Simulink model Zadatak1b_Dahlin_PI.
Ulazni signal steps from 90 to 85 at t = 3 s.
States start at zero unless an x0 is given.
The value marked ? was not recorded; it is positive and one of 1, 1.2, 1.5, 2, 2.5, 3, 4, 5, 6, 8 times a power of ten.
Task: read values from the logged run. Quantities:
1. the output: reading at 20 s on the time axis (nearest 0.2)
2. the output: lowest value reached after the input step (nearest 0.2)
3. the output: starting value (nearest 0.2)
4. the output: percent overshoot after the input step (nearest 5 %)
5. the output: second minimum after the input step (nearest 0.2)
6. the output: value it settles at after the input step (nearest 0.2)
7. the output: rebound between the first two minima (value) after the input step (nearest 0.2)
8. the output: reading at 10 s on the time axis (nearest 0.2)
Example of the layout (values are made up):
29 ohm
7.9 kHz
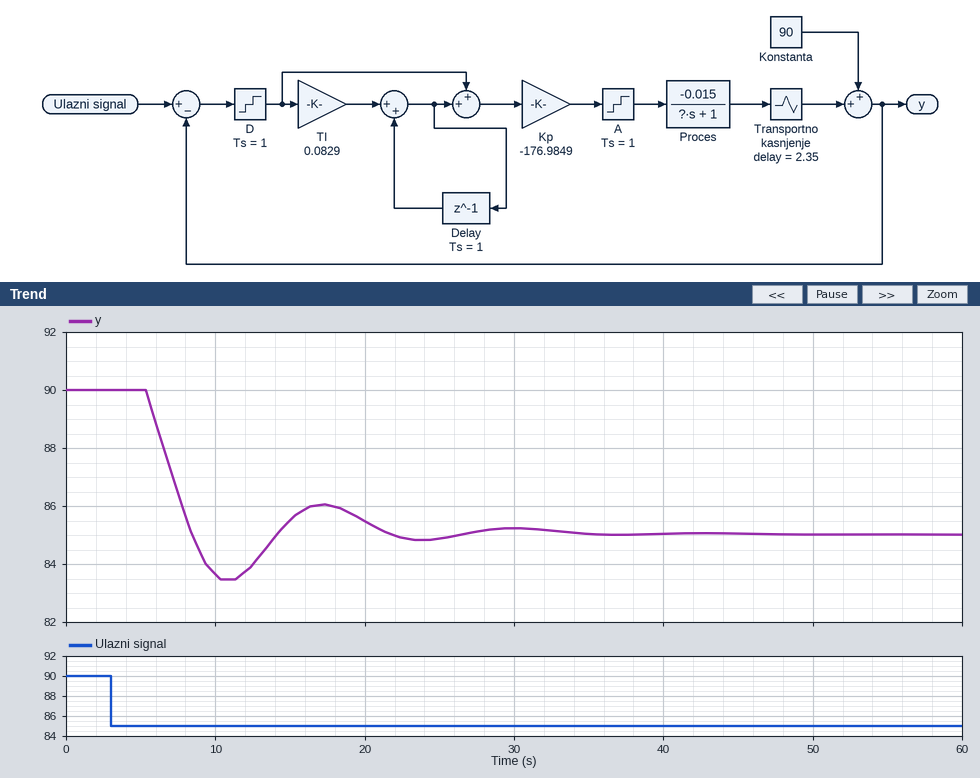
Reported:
85.4
83.4
90.0
30 %
84.8
85.0
86.0
83.6
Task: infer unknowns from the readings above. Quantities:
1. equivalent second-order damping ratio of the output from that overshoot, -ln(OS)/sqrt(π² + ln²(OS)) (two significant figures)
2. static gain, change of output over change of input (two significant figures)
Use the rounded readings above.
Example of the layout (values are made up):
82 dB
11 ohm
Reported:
0.36
1.0
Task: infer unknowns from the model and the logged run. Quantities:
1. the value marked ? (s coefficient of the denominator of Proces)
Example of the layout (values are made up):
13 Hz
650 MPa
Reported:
8
